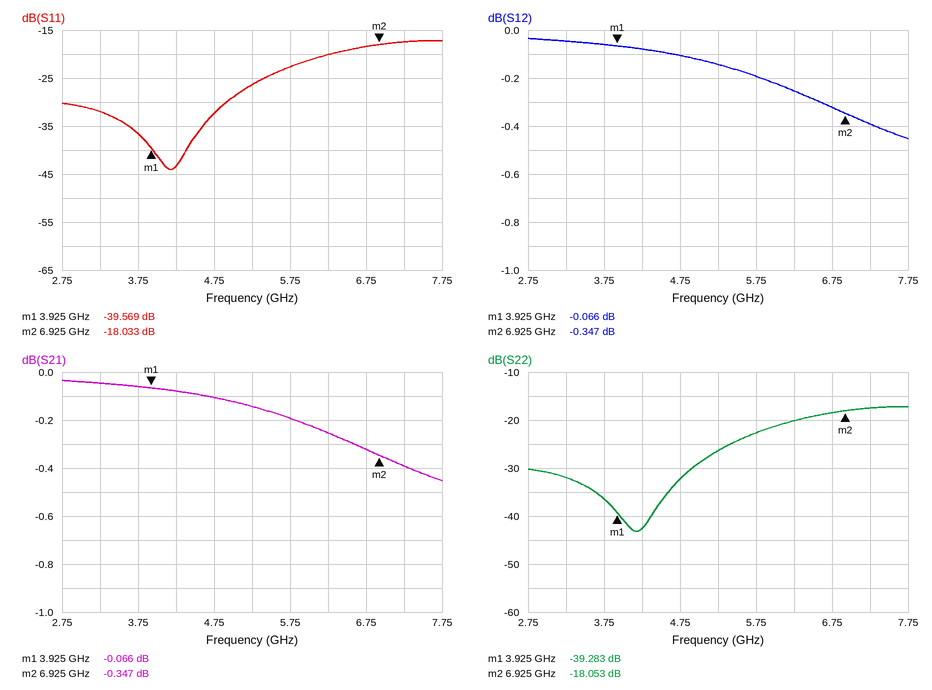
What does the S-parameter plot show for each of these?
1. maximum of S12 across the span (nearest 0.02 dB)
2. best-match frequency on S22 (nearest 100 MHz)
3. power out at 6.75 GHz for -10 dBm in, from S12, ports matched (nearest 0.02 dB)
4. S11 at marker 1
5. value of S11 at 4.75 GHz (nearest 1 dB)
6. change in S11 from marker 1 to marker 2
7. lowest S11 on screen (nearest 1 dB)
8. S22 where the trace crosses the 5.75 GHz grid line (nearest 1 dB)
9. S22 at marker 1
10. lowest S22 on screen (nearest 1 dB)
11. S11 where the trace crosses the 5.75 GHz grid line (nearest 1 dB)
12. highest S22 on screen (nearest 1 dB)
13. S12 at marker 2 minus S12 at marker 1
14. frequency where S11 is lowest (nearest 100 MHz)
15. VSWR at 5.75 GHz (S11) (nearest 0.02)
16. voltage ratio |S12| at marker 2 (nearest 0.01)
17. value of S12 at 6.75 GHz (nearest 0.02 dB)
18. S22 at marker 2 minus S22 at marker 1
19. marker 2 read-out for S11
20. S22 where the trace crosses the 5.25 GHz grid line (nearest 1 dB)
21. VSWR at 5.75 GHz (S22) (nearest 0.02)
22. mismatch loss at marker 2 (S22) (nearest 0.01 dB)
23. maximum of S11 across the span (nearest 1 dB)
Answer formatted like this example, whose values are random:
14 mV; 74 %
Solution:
-0.04 dB; 4.2 GHz; -10.32 dBm; -39.569 dB; -32 dB; 21.536 dB; -44 dB; -23 dB; -39.283 dB; -43 dB; -23 dB; -17 dB; -0.281 dB; 4.2 GHz; 1.16; 0.96; -0.32 dB; 21.230 dB; -18.033 dB; -26 dB; 1.16; 0.07 dB; -17 dB
